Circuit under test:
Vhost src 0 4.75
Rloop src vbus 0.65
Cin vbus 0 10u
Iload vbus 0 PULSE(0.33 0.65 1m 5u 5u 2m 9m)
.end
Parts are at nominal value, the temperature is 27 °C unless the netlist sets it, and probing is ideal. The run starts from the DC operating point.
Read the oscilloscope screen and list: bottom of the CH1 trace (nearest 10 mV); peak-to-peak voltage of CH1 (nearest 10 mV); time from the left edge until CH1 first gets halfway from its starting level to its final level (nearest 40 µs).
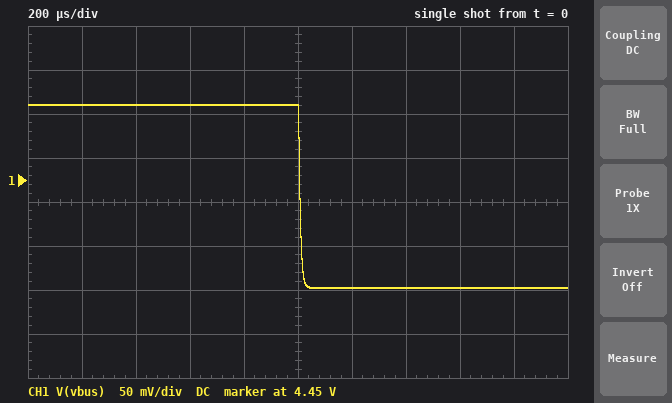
4.33 V
210 mV
1.00 ms
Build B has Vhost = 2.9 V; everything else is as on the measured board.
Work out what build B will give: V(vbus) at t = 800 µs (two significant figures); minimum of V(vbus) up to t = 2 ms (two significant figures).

2.7 V
2.5 V
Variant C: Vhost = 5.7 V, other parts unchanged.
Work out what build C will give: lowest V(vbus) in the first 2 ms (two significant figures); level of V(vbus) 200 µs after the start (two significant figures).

5.3 V
5.5 V
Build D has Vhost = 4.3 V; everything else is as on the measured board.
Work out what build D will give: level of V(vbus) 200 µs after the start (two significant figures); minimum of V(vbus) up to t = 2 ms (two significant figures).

4.1 V
3.9 V
